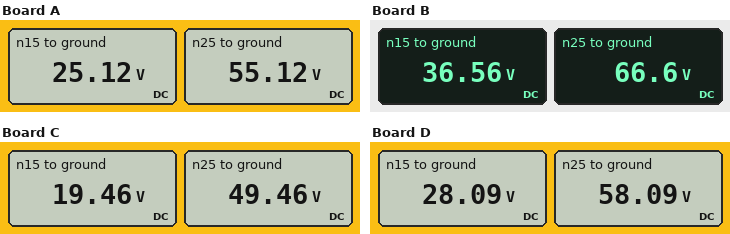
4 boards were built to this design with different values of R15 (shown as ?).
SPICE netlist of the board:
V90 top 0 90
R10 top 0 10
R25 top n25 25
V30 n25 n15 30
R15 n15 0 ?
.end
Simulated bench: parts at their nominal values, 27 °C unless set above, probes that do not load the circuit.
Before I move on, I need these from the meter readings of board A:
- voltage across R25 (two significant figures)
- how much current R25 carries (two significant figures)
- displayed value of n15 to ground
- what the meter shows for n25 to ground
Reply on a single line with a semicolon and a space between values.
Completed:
35 V; 1.4 A; 25.12 V; 55.12 V
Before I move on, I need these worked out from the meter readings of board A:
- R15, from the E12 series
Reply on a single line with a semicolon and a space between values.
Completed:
18 Ω
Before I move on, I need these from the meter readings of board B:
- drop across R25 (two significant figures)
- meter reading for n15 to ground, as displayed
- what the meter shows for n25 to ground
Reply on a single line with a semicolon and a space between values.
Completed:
23 V; 36.56 V; 66.6 V
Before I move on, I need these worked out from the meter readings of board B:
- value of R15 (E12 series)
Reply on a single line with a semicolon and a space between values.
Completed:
39 Ω
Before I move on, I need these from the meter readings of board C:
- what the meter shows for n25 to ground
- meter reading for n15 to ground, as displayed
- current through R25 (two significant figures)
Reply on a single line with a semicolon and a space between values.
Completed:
49.46 V; 19.46 V; 1.6 A
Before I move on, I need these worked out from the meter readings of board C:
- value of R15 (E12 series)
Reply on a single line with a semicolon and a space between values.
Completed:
12 Ω
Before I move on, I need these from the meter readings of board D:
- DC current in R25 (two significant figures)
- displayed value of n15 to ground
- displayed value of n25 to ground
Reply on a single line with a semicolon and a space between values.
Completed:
1.3 A; 28.09 V; 58.09 V
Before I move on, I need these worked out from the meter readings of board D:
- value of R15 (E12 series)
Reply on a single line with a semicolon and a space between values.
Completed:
22 Ω
